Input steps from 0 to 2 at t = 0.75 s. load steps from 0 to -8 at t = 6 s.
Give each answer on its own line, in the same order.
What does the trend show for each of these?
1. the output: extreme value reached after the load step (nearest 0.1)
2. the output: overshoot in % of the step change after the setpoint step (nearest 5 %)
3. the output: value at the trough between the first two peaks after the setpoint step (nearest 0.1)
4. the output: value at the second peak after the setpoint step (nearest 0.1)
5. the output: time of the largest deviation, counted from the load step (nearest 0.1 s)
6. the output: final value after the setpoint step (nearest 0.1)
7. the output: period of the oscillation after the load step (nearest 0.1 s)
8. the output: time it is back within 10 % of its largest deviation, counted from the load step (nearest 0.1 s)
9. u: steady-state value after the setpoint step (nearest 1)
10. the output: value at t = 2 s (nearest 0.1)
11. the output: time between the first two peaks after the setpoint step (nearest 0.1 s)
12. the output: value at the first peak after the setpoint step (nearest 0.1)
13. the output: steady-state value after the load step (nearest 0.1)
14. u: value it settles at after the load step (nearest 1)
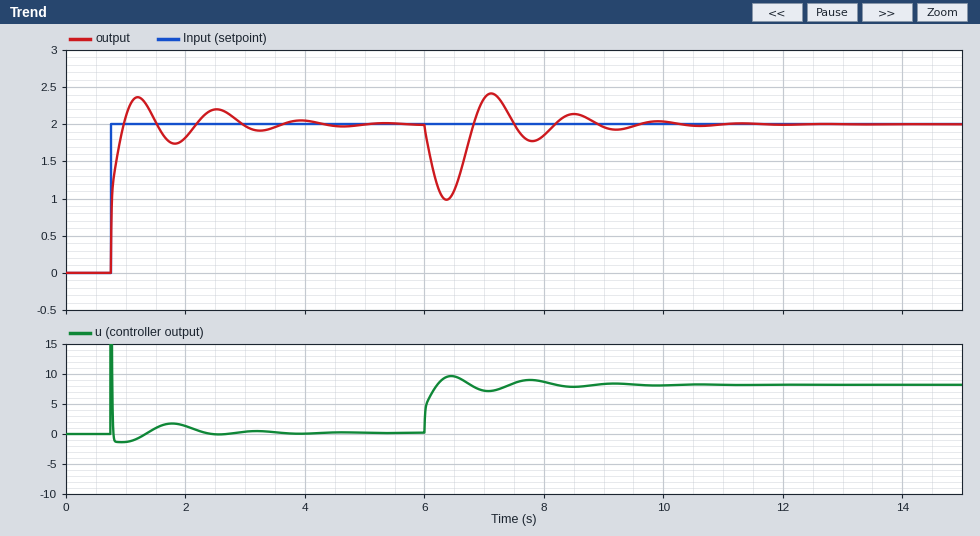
1.0
20 %
1.7
2.2
0.4 s
2.0
1.4 s
2.7 s
0
1.8
1.3 s
2.4
2.0
8
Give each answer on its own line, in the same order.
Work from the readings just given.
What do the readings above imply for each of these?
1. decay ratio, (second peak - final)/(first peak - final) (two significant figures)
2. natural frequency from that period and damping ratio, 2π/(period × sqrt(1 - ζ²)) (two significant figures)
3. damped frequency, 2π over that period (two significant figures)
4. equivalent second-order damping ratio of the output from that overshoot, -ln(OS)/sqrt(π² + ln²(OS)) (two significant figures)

0.50
5.4 rad/s
4.8 rad/s
0.46
